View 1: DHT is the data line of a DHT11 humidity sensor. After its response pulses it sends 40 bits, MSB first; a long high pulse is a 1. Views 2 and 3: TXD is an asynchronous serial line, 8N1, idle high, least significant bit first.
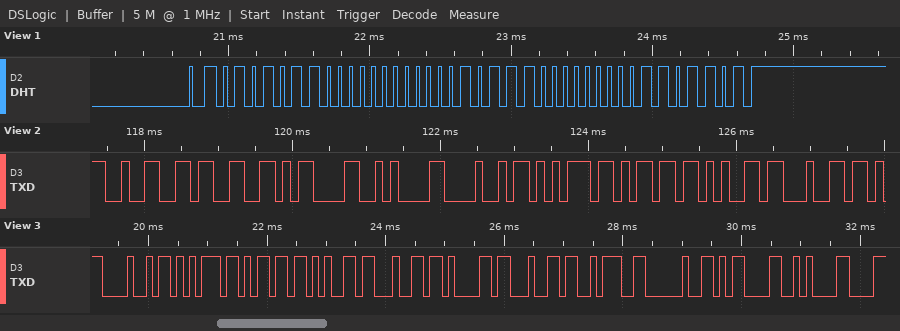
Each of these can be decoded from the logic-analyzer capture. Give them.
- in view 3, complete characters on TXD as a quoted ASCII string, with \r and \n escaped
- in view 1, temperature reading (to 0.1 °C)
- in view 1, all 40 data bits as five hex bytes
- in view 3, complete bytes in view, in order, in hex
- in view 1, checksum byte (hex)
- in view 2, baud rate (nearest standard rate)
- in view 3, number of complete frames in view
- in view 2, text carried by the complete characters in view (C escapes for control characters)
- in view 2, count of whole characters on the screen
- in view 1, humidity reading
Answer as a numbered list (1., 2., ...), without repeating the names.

1. "Humedad: \r\n"
2. 23.0 °C
3. 56 00 17 00 6D
4. 48 75 6D 65 64 61 64 3A 20 0D 0A
5. 0x6D
6. 9600 baud
7. 11
8. "23\r\nHumed"
9. 9
10. 86 %
